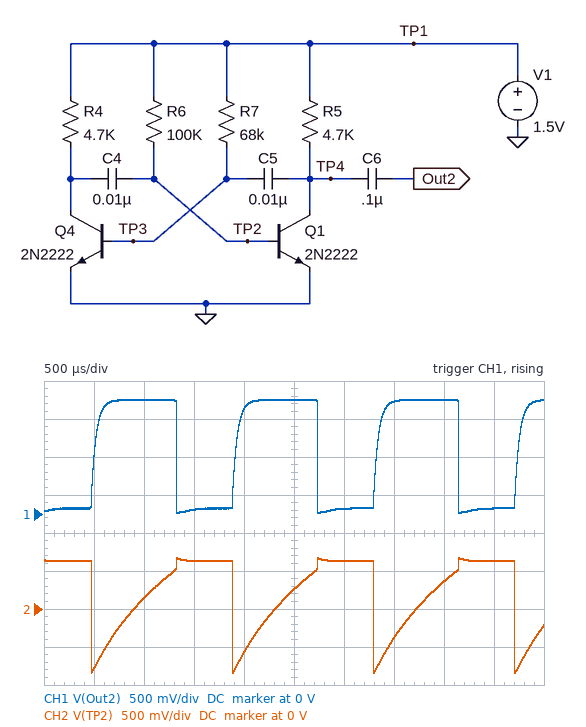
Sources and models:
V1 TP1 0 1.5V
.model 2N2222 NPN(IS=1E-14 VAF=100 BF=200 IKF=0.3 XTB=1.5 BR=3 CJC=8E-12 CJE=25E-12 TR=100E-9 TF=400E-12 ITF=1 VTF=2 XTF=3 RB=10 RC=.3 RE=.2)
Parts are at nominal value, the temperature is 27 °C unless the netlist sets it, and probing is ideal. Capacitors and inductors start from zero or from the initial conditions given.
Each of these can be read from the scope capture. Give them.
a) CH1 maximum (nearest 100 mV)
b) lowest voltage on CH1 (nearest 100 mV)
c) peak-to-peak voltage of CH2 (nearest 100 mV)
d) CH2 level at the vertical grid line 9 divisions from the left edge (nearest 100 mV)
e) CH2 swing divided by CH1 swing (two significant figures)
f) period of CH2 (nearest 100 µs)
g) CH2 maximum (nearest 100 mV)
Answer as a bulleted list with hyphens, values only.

- 1.5 V
- 0 V
- 1.5 V
- 600 mV
- 1.0
- 1.4 ms
- 700 mV
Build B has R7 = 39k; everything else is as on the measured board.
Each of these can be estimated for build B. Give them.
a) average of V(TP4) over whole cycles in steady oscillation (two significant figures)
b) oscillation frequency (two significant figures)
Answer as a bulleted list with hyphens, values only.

- 1.1 V
- 840 Hz
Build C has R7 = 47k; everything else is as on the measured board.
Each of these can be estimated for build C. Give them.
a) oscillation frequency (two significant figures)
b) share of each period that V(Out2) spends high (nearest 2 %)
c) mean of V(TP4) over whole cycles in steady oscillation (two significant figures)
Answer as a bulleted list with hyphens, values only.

- 800 Hz
- 68 %
- 1.0 V
